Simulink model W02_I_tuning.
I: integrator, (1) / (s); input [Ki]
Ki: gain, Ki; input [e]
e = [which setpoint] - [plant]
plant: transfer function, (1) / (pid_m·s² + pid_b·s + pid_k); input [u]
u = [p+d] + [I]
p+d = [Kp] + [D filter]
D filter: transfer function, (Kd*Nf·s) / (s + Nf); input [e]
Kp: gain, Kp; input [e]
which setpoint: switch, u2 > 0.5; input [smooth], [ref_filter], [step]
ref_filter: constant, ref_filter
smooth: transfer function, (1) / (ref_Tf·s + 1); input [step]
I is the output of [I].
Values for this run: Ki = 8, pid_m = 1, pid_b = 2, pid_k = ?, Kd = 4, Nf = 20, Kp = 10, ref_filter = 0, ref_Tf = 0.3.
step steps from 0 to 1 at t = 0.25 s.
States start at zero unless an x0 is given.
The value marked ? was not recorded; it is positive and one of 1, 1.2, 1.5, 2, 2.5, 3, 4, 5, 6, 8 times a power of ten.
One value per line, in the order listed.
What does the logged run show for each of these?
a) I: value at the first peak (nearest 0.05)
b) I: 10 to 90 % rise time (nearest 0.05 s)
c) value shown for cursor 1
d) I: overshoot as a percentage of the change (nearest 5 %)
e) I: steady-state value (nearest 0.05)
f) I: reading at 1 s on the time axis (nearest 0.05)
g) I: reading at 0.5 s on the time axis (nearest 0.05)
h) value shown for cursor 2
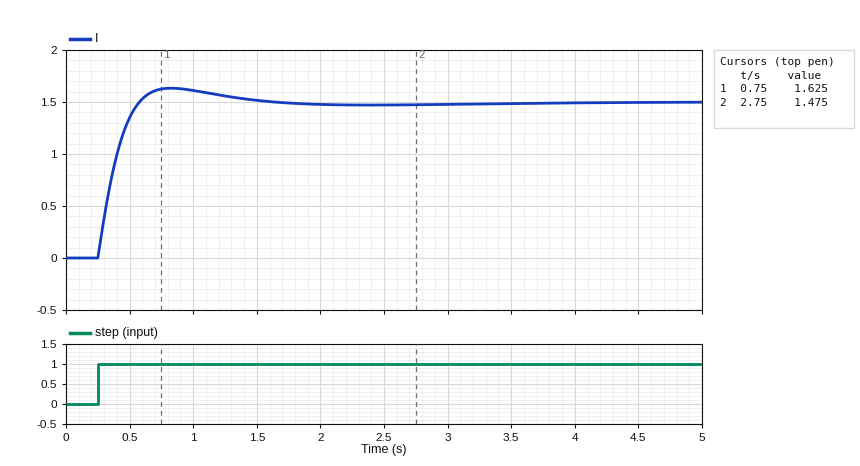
1.65
0.25 s
1.625
10 %
1.50
1.60
1.35
1.475
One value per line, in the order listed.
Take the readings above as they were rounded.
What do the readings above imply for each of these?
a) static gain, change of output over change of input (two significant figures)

1.5
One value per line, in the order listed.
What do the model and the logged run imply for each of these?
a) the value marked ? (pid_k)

1.5
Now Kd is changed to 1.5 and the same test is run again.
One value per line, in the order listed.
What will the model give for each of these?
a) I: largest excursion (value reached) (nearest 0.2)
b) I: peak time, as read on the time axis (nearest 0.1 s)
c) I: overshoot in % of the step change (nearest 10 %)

2.2
0.8 s
50 %
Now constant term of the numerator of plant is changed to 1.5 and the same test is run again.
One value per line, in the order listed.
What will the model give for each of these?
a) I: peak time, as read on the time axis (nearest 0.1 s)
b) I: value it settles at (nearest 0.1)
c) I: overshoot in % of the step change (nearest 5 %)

0.6 s
1.0
15 %
